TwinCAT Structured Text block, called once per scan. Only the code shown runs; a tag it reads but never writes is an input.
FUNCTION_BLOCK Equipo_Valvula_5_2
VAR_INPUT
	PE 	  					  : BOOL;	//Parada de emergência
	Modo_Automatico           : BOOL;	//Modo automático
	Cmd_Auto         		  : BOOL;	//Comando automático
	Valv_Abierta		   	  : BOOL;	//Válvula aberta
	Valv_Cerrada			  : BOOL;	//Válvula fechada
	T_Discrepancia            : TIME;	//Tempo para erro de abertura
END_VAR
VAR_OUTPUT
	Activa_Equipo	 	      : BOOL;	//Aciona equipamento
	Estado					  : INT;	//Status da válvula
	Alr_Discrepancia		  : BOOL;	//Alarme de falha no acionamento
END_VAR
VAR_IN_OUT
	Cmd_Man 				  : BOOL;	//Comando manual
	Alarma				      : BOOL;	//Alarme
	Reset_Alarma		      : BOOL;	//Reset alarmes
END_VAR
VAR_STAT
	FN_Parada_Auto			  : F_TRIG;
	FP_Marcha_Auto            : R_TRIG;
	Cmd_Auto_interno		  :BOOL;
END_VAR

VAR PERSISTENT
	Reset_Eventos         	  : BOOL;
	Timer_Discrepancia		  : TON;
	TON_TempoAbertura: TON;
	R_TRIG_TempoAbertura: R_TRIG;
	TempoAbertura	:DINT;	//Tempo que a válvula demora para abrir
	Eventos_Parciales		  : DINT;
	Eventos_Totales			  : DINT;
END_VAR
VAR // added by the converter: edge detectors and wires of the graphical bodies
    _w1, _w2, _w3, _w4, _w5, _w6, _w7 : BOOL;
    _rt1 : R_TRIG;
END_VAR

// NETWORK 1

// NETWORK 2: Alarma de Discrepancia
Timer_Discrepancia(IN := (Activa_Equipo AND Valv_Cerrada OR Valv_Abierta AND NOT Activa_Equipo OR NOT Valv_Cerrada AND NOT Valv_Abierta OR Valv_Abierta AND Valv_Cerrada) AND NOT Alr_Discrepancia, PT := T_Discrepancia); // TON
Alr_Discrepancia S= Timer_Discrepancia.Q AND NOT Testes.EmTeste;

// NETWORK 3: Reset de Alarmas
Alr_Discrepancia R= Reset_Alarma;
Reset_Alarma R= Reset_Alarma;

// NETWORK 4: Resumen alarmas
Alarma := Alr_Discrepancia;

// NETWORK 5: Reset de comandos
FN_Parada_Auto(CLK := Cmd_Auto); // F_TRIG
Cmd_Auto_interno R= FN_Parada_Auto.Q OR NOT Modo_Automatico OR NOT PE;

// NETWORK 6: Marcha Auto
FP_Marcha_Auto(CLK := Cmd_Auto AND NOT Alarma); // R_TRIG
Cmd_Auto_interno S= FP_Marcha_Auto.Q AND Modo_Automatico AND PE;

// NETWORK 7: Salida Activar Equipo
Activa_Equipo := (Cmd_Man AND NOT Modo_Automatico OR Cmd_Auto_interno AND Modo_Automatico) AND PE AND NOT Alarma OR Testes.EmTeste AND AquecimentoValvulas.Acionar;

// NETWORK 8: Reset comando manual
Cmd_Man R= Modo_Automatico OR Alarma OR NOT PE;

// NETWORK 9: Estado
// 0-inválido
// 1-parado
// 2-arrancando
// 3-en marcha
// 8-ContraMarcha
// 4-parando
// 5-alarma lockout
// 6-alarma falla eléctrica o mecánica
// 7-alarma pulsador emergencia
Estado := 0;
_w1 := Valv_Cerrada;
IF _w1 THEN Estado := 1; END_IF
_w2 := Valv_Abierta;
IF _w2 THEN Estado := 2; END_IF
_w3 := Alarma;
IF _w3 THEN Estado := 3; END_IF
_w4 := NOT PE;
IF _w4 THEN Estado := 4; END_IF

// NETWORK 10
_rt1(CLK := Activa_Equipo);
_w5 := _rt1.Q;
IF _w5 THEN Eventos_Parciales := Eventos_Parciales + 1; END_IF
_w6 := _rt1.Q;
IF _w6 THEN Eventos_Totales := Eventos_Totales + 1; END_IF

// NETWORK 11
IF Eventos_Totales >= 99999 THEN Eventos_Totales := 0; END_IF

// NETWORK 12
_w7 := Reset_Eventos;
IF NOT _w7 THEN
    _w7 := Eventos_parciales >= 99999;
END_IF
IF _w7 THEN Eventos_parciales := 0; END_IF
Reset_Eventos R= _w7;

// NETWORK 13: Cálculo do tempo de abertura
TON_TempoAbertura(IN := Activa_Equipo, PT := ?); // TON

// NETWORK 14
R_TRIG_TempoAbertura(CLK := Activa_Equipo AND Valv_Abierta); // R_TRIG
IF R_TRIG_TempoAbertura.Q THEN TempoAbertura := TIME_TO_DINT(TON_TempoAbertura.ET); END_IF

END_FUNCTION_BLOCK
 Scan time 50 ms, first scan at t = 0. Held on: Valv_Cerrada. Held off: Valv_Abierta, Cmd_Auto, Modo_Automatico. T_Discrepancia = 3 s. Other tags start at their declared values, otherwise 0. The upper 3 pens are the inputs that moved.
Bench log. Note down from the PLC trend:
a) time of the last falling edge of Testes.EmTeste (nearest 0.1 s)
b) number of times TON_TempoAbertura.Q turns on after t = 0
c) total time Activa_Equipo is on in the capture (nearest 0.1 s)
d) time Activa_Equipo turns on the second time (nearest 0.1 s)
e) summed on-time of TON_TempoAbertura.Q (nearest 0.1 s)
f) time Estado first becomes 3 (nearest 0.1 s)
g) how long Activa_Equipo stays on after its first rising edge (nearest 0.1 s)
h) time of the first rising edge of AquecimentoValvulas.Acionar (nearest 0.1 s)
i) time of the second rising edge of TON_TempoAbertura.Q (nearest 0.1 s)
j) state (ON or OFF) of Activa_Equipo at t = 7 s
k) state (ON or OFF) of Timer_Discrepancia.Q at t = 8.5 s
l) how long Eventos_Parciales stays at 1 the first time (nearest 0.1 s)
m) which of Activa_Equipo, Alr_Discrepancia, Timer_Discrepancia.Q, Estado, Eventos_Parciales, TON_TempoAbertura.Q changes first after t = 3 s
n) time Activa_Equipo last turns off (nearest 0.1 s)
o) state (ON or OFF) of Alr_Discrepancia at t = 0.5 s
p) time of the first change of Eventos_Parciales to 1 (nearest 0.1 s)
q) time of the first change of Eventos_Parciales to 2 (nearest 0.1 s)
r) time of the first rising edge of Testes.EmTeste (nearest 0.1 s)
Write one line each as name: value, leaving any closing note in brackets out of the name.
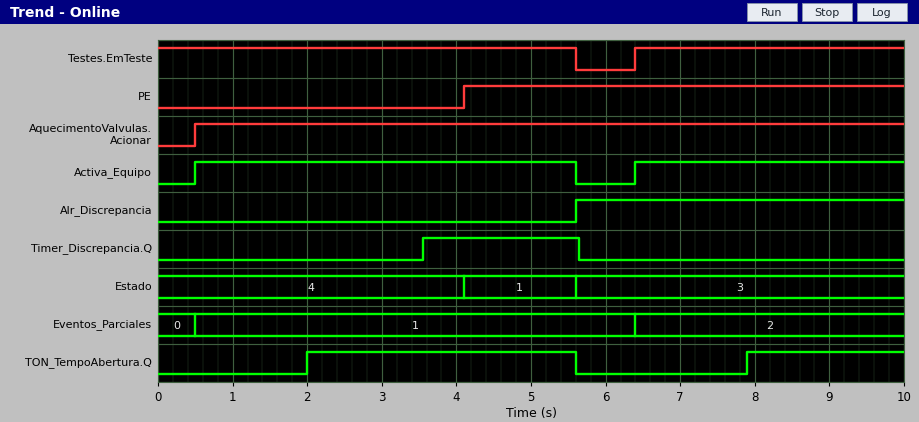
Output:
time of the last falling edge of Testes.EmTeste: 5.6 s
number of times TON_TempoAbertura.Q turns on after t = 0: 2
total time Activa_Equipo is on in the capture: 8.7 s
time Activa_Equipo turns on the second time: 6.4 s
summed on-time of TON_TempoAbertura.Q: 5.7 s
time Estado first becomes 3: 5.6 s
how long Activa_Equipo stays on after its first rising edge: 5.1 s
time of the first rising edge of AquecimentoValvulas.Acionar: 0.5 s
time of the second rising edge of TON_TempoAbertura.Q: 7.9 s
state (ON or OFF) of Activa_Equipo at t = 7 s: ON
state (ON or OFF) of Timer_Discrepancia.Q at t = 8.5 s: OFF
how long Eventos_Parciales stays at 1 the first time: 5.9 s
which of Activa_Equipo, Alr_Discrepancia, Timer_Discrepancia.Q, Estado, Eventos_Parciales, TON_TempoAbertura.Q changes first after t = 3 s: Timer_Discrepancia.Q
time Activa_Equipo last turns off: 5.6 s
state (ON or OFF) of Alr_Discrepancia at t = 0.5 s: OFF
time of the first change of Eventos_Parciales to 1: 0.5 s
time of the first change of Eventos_Parciales to 2: 6.4 s
time of the first rising edge of Testes.EmTeste: 6.4 s
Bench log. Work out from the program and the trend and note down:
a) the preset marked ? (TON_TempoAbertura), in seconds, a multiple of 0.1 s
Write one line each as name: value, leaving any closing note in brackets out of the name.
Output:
the preset marked ? (TON_TempoAbertura), in seconds, a multiple of 0.1 s: 1.5 s
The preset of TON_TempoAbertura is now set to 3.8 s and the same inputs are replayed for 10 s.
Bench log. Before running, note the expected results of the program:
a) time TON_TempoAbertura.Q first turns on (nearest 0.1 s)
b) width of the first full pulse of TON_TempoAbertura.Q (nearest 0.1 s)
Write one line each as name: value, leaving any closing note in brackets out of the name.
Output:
time TON_TempoAbertura.Q first turns on: 4.3 s
width of the first full pulse of TON_TempoAbertura.Q: 1.3 s
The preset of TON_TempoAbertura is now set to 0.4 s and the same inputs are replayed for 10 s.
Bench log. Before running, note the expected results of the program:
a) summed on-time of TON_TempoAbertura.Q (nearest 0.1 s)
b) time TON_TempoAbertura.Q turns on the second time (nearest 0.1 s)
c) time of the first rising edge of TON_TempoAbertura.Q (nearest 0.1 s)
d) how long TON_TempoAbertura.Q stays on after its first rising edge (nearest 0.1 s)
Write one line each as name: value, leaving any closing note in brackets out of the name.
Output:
summed on-time of TON_TempoAbertura.Q: 7.9 s
time TON_TempoAbertura.Q turns on the second time: 6.8 s
time of the first rising edge of TON_TempoAbertura.Q: 0.9 s
how long TON_TempoAbertura.Q stays on after its first rising edge: 4.7 s
